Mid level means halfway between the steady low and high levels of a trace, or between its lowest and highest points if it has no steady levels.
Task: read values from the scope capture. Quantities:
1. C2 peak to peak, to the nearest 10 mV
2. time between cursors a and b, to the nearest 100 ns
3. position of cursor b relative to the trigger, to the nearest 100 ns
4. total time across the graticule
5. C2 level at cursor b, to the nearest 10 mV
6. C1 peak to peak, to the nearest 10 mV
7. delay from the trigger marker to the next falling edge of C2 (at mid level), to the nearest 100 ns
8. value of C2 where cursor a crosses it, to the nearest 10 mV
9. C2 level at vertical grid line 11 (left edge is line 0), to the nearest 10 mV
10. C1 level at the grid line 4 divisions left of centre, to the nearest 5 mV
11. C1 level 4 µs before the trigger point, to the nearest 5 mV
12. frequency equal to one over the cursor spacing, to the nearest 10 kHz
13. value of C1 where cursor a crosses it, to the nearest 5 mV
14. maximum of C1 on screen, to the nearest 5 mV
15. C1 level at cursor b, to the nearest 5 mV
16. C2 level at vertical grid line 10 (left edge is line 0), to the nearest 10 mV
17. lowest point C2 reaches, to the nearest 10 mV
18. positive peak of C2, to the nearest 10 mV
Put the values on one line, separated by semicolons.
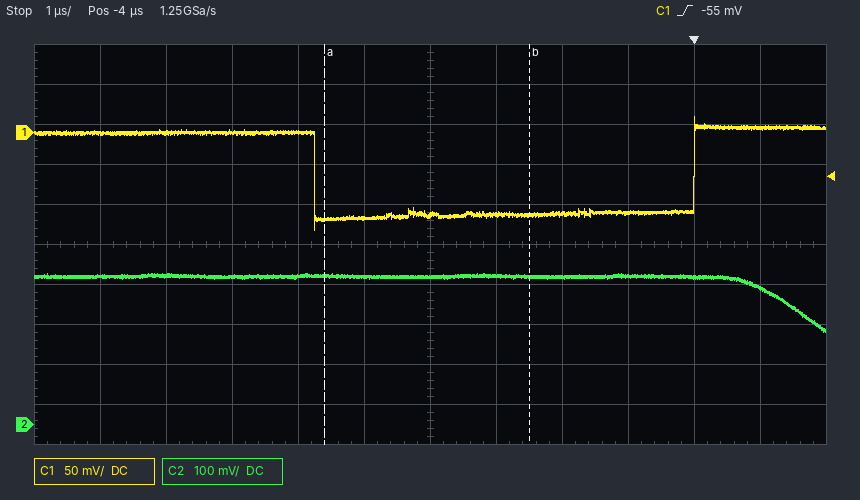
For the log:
150 mV; 3.1 µs; -2.5 µs; 12 µs; 370 mV; 140 mV; 1.4 µs; 370 mV; 340 mV; 0 mV; -105 mV; 320 kHz; -110 mV; 20 mV; -105 mV; 370 mV; 230 mV; 380 mV
